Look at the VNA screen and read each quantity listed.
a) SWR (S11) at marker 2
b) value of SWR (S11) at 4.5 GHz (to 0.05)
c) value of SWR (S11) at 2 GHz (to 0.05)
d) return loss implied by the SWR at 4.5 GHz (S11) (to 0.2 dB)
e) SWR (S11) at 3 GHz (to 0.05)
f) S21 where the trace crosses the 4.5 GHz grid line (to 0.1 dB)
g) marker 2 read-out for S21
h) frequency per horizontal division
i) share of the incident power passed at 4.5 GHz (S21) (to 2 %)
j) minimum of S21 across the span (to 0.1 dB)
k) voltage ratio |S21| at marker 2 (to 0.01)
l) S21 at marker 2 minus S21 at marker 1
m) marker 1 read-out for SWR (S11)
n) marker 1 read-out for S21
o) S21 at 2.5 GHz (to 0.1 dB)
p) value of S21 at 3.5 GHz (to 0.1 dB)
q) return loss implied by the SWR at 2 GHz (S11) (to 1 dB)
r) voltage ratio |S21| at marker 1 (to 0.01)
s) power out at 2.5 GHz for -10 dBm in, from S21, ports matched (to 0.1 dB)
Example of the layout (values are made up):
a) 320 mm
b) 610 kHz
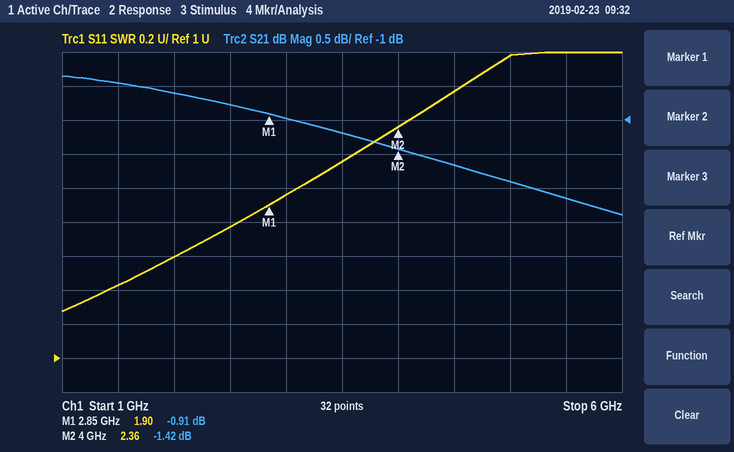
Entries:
a) 2.36
b) 2.55
c) 1.60
d) 7.2 dB
e) 1.95
f) -1.7 dB
g) -1.42 dB
h) 500 MHz
i) 68 %
j) -2.4 dB
k) 0.85
l) -0.51 dB
m) 1.90
n) -0.91 dB
o) -0.8 dB
p) -1.2 dB
q) 13 dB
r) 0.90
s) -10.8 dBm
